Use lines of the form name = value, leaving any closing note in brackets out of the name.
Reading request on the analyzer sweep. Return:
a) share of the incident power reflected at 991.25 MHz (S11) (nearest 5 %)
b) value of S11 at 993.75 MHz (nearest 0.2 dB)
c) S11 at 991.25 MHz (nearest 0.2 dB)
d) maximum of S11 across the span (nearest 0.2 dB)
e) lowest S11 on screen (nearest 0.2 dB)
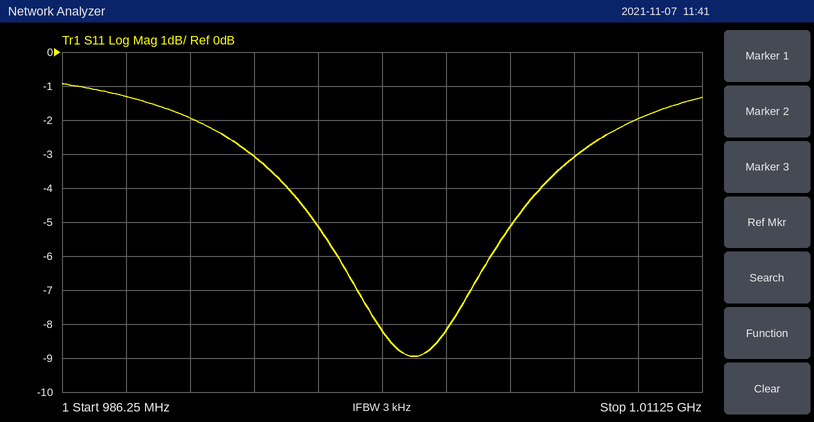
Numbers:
share of the incident power reflected at 991.25 MHz (S11) = 65 %
value of S11 at 993.75 MHz = -3.0 dB
S11 at 991.25 MHz = -2.0 dB
maximum of S11 across the span = -1.0 dB
lowest S11 on screen = -9.0 dB
